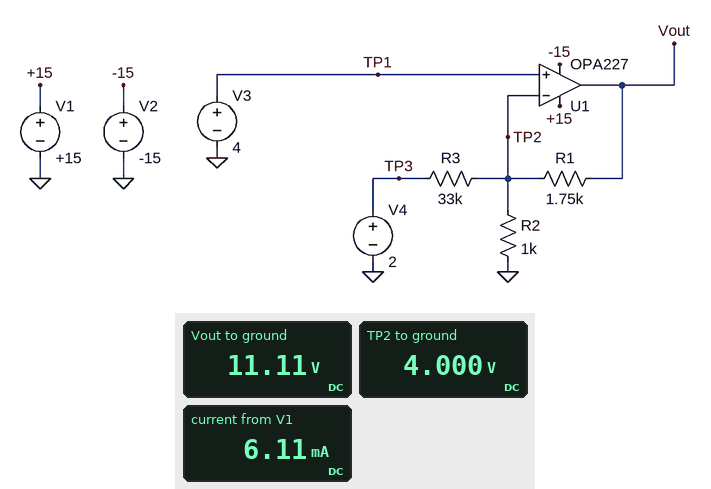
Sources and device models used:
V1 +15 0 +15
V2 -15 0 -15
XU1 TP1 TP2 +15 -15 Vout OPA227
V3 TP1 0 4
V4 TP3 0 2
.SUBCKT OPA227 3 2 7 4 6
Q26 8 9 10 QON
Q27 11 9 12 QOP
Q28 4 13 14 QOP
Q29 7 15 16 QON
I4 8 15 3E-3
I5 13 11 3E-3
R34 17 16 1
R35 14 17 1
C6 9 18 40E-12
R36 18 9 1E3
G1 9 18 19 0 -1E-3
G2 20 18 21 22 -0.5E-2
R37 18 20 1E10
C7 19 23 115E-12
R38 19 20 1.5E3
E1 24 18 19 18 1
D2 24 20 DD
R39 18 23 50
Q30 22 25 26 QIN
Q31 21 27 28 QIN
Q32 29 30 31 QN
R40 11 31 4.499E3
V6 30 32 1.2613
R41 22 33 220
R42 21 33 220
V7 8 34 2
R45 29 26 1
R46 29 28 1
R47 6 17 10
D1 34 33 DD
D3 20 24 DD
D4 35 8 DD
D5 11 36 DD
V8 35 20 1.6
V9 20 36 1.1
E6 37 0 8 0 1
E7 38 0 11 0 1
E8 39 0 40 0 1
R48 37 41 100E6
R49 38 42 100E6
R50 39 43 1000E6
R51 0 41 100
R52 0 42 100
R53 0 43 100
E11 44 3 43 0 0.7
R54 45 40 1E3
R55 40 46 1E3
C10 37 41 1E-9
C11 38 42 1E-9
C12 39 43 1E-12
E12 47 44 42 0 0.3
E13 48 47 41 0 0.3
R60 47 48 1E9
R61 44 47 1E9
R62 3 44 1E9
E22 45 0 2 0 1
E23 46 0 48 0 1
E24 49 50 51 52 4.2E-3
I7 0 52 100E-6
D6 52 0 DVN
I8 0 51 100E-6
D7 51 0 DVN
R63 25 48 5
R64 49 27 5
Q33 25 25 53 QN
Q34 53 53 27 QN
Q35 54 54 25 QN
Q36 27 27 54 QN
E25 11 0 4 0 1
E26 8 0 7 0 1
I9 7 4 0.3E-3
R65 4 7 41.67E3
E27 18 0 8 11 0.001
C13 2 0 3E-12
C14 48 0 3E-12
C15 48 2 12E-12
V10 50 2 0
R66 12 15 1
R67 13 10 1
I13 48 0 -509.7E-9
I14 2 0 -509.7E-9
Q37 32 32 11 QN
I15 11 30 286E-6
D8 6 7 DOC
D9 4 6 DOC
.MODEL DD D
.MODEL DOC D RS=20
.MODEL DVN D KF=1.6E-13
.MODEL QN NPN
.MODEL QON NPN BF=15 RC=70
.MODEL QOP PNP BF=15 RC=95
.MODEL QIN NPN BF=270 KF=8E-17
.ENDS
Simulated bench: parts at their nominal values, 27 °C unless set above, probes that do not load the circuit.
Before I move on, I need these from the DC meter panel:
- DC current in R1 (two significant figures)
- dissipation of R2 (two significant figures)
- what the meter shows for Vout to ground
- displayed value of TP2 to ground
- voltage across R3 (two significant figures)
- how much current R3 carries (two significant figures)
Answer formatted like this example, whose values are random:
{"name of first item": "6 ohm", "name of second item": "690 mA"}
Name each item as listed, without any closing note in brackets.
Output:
{"DC current in R1": "4.1 mA", "dissipation of R2": "16 mW", "what the meter shows for Vout to ground": "11.11 V", "displayed value of TP2 to ground": "4.000 V", "voltage across R3": "2.0 V", "how much current R3 carries": "61 µA"}
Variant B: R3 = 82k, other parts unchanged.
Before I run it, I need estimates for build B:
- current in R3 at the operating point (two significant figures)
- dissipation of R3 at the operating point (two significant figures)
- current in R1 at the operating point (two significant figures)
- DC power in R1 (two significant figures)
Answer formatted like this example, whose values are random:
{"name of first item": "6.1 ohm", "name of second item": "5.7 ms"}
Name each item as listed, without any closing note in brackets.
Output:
{"current in R3 at the operating point": "24 µA", "dissipation of R3 at the operating point": "49 µW", "current in R1 at the operating point": "4.0 mA", "DC power in R1": "28 mW"}
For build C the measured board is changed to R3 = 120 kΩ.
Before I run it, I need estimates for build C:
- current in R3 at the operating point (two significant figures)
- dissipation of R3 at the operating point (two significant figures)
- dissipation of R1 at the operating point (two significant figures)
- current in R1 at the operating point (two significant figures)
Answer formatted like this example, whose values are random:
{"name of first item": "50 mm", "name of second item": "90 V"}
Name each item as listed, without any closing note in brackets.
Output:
{"current in R3 at the operating point": "17 µA", "dissipation of R3 at the operating point": "33 µW", "dissipation of R1 at the operating point": "28 mW", "current in R1 at the operating point": "4.0 mA"}
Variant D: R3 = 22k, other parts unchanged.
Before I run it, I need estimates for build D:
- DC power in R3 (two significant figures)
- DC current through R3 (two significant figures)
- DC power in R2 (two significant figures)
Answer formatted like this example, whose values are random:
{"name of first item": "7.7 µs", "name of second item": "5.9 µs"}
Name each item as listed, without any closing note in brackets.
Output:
{"DC power in R3": "180 µW", "DC current through R3": "91 µA", "DC power in R2": "16 mW"}
